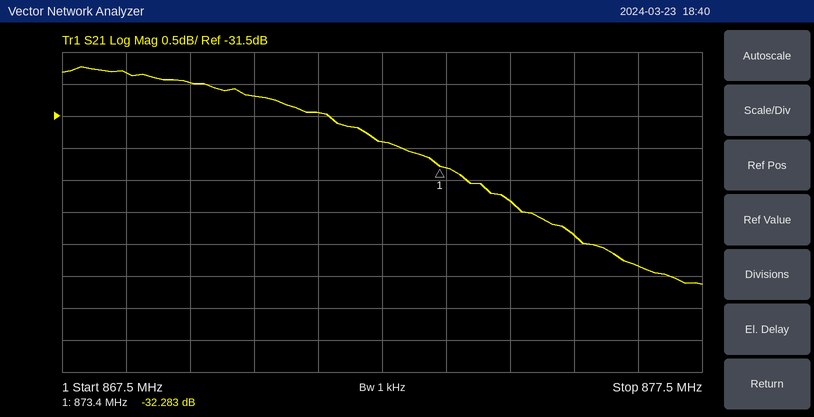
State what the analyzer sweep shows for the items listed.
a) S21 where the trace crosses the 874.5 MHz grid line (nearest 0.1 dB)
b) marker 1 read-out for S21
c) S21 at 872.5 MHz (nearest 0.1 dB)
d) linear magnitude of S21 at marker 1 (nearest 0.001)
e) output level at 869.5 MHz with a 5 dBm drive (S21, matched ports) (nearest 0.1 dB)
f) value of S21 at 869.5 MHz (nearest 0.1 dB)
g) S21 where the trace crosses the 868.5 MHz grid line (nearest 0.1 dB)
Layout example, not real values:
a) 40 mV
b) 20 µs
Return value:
a) -32.8 dB
b) -32.283 dB
c) -31.9 dB
d) 0.024
e) -26.0 dBm
f) -31.0 dB
g) -30.8 dB
